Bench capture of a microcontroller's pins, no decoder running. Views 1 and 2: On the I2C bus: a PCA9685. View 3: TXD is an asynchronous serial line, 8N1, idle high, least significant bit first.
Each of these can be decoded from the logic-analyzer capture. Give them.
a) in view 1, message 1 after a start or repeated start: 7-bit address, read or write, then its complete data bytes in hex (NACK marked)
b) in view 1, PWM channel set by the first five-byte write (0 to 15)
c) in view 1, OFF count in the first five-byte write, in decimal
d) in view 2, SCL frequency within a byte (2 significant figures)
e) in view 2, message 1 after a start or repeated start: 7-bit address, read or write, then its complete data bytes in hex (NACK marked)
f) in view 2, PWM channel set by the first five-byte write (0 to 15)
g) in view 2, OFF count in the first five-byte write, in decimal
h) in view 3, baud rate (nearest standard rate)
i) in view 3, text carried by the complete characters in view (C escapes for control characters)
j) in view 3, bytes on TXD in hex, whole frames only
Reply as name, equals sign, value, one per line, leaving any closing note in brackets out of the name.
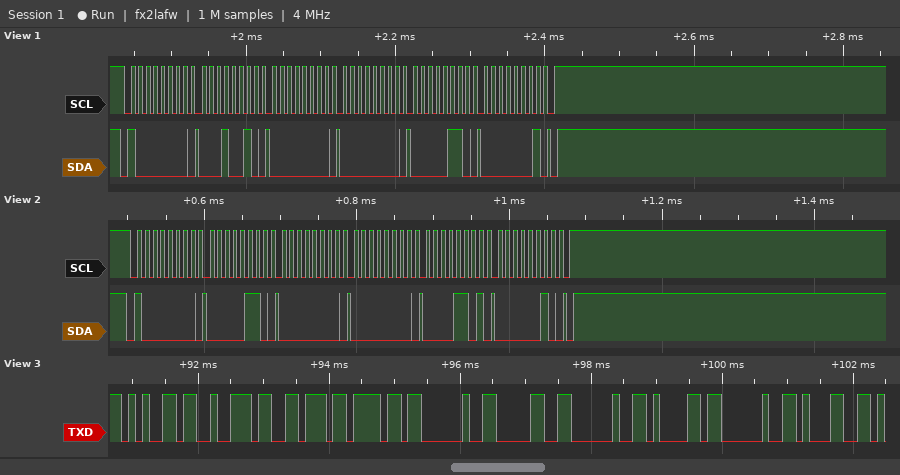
in view 1, message 1 after a start or repeated start: 7-bit address, read or write, then its complete data bytes in hex = 0x40 write: 12 00 00 06 01
in view 1, PWM channel set by the first five-byte write = 3
in view 1, OFF count in the first five-byte write, in decimal = 262
in view 2, SCL frequency within a byte = 100 kHz
in view 2, message 1 after a start or repeated start: 7-bit address, read or write, then its complete data bytes in hex = 0x40 write: 06 00 00 0D 02
in view 2, PWM channel set by the first five-byte write = 0
in view 2, OFF count in the first five-byte write, in decimal = 525
in view 3, baud rate = 9600 baud
in view 3, text carried by the complete characters in view = "ervo 0 a 1"
in view 3, bytes on TXD in hex, whole frames only = 0x65 0x72 0x76 0x6F 0x20 0x30 0x20 0x61 0x20 0x31
